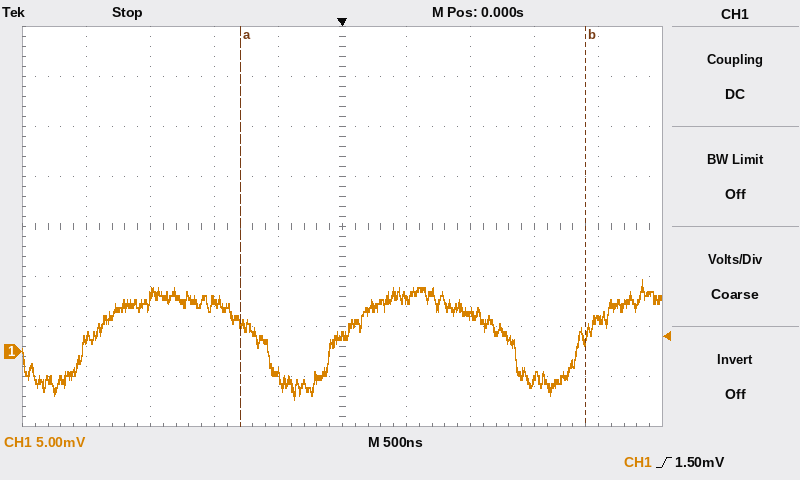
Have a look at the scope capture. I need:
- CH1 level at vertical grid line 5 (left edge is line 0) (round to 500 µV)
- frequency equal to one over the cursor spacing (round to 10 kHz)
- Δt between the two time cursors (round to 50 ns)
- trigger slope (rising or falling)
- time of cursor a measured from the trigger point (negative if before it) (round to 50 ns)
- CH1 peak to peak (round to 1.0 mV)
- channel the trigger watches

1.5 mV
370 kHz
2.70 µs
rising
-800 ns
12.0 mV
CH1
